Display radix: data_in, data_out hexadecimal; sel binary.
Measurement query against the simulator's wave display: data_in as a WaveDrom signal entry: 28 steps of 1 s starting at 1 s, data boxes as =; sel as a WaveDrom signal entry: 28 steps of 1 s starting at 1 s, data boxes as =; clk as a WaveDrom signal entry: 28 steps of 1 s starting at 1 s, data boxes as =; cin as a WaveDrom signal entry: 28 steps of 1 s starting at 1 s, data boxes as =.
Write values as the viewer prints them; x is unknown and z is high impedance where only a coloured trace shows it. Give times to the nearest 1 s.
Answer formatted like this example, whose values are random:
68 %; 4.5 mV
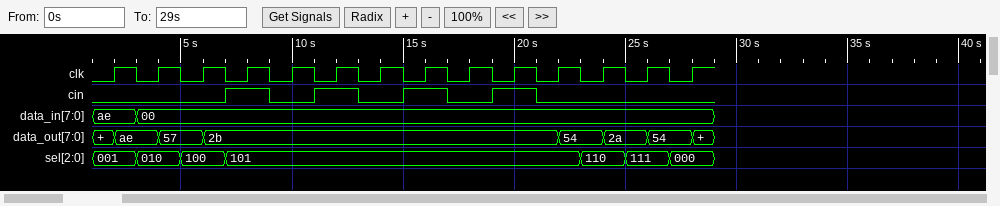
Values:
{name: 'data_in', wave: '=.=.........................', data: 'ae 00'}; {name: 'sel', wave: '=.=.=.=...............=.=.=.', data: '001 010 100 101 110 111 000'}; {name: 'clk', wave: '0101010101010101010101010101'}; {name: 'cin', wave: '0.....1.0.1.0.1.0.1.0.......'}
